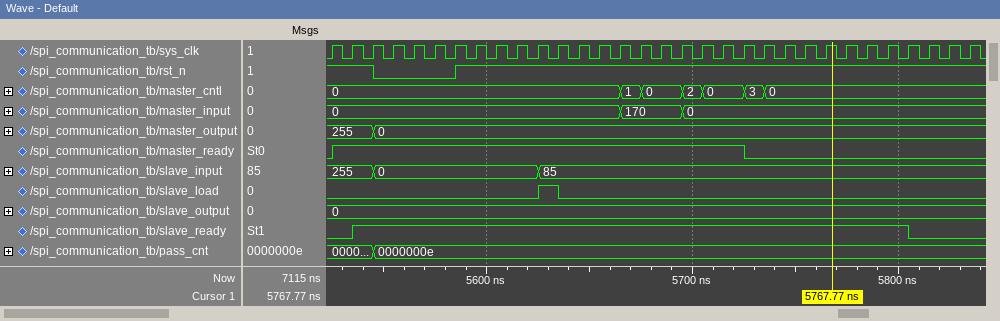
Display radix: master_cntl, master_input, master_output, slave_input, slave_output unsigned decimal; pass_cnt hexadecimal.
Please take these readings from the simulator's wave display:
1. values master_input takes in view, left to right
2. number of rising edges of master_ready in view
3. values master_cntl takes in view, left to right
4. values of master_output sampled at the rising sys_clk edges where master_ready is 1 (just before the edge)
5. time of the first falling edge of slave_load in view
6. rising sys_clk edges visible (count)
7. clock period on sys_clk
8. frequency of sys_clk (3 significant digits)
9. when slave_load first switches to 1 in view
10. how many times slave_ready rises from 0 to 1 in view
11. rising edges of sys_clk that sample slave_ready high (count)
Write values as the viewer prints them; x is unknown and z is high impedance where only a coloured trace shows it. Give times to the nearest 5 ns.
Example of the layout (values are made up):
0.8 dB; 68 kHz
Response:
0, 170, 0; 1; 0, 1, 0, 2, 0, 3, 0; 255, 255, 0, 0, 0, 0, 0, 0, 0, 0, 0, 0, 0, 0, 0, 0, 0, 0, 0, 0; 5635 ns; 32; 10 ns; 100 MHz; 5625 ns; 1; 27
